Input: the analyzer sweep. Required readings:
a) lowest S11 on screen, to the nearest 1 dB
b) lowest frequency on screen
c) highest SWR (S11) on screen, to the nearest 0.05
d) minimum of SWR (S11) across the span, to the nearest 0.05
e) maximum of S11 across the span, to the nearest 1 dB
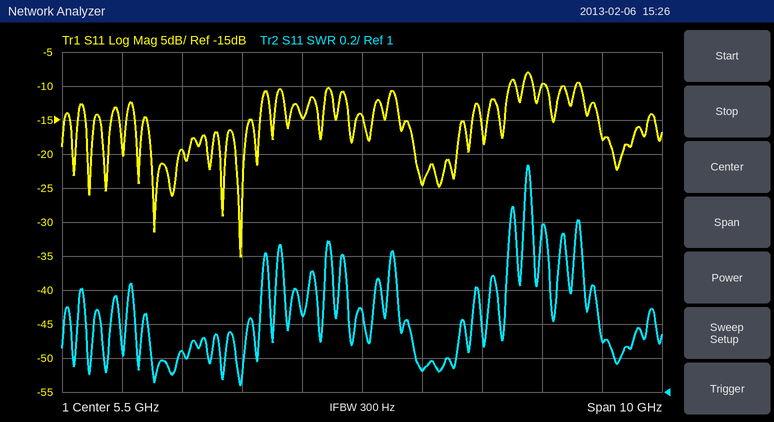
-35 dB
500 MHz
2.35
1.05
-8 dB
